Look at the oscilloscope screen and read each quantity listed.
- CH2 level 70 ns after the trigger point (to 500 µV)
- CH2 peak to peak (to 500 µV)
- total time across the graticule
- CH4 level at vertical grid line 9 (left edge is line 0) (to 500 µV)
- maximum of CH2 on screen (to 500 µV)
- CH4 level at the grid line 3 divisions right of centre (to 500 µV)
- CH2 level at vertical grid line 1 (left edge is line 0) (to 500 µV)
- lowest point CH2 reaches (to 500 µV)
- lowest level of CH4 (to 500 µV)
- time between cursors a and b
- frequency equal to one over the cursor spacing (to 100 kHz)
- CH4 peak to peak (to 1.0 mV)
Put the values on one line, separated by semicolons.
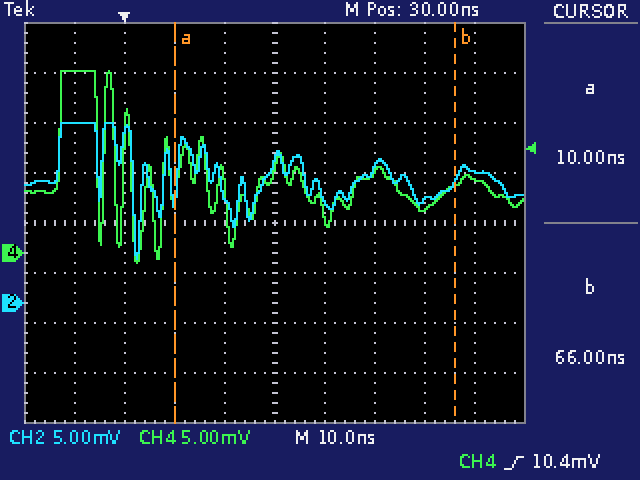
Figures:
13.0 mV; 13.5 mV; 100 ns; 7.5 mV; 18.0 mV; 4.5 mV; 18.0 mV; 4.5 mV; -1.0 mV; 56 ns; 17.9 MHz; 19.0 mV
